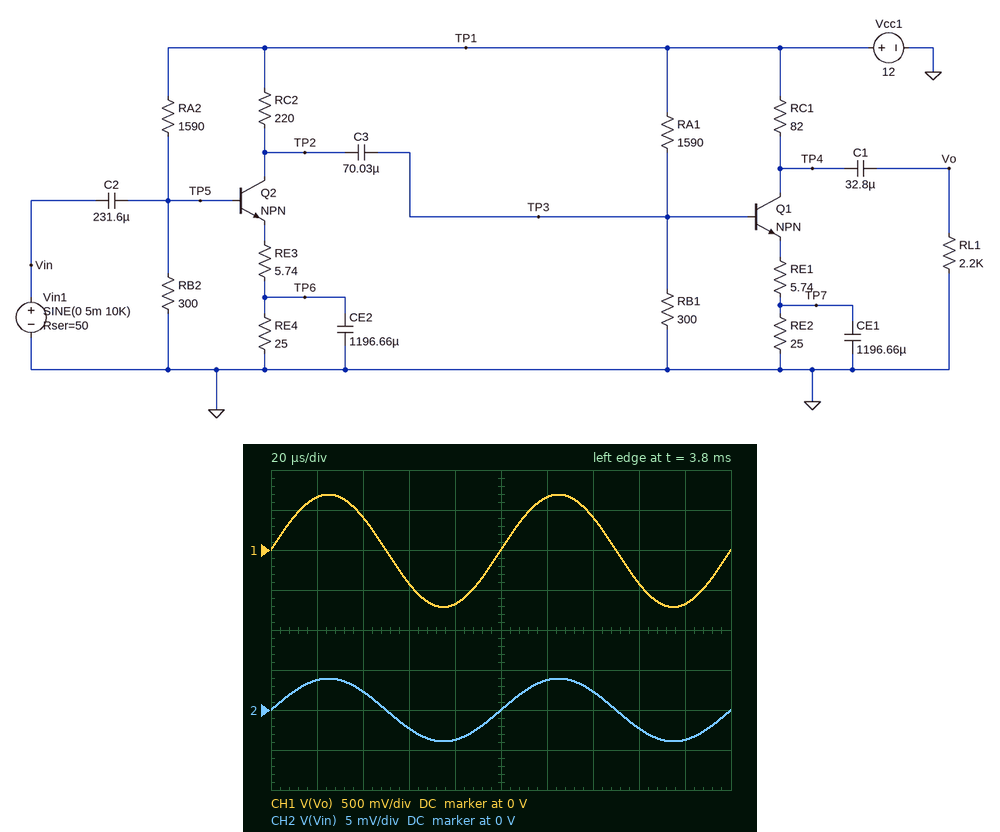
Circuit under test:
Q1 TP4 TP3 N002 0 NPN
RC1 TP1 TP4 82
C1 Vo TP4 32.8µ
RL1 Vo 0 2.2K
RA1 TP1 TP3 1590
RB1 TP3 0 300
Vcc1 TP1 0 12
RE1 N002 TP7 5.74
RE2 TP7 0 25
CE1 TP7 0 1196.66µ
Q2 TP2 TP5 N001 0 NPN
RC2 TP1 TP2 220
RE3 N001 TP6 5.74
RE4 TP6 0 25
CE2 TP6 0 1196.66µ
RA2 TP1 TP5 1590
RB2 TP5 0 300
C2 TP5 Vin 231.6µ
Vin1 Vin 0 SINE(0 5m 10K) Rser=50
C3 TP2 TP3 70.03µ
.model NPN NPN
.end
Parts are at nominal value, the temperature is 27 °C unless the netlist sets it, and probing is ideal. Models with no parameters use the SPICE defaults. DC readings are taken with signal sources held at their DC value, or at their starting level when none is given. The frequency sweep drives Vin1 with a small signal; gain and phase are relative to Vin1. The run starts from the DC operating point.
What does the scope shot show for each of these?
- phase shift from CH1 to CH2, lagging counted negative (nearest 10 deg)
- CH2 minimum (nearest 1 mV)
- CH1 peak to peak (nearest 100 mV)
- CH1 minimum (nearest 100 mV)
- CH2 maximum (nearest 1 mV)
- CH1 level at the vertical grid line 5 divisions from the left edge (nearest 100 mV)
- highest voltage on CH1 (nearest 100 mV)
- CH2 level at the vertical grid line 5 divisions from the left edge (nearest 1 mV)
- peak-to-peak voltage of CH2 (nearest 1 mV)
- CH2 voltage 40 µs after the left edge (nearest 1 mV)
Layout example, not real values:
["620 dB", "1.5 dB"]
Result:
["0 deg", "-4 mV", "1.4 V", "-700 mV", "4 mV", "0 V", "700 mV", "0 V", "8 mV", "2 mV"]
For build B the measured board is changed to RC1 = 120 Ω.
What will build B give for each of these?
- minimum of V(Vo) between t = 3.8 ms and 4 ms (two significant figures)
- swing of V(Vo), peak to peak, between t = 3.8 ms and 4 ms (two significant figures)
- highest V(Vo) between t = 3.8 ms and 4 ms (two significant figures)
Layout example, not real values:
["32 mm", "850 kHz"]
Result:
["-1.0 V", "2.0 V", "1.0 V"]
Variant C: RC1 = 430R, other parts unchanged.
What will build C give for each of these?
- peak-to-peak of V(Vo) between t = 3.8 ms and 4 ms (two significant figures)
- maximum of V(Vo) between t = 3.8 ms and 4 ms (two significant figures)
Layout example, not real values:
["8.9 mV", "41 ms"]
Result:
["58 mV", "45 mV"]
